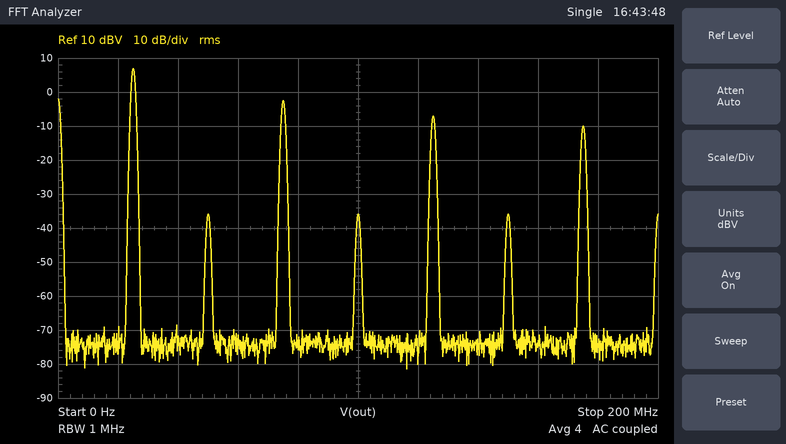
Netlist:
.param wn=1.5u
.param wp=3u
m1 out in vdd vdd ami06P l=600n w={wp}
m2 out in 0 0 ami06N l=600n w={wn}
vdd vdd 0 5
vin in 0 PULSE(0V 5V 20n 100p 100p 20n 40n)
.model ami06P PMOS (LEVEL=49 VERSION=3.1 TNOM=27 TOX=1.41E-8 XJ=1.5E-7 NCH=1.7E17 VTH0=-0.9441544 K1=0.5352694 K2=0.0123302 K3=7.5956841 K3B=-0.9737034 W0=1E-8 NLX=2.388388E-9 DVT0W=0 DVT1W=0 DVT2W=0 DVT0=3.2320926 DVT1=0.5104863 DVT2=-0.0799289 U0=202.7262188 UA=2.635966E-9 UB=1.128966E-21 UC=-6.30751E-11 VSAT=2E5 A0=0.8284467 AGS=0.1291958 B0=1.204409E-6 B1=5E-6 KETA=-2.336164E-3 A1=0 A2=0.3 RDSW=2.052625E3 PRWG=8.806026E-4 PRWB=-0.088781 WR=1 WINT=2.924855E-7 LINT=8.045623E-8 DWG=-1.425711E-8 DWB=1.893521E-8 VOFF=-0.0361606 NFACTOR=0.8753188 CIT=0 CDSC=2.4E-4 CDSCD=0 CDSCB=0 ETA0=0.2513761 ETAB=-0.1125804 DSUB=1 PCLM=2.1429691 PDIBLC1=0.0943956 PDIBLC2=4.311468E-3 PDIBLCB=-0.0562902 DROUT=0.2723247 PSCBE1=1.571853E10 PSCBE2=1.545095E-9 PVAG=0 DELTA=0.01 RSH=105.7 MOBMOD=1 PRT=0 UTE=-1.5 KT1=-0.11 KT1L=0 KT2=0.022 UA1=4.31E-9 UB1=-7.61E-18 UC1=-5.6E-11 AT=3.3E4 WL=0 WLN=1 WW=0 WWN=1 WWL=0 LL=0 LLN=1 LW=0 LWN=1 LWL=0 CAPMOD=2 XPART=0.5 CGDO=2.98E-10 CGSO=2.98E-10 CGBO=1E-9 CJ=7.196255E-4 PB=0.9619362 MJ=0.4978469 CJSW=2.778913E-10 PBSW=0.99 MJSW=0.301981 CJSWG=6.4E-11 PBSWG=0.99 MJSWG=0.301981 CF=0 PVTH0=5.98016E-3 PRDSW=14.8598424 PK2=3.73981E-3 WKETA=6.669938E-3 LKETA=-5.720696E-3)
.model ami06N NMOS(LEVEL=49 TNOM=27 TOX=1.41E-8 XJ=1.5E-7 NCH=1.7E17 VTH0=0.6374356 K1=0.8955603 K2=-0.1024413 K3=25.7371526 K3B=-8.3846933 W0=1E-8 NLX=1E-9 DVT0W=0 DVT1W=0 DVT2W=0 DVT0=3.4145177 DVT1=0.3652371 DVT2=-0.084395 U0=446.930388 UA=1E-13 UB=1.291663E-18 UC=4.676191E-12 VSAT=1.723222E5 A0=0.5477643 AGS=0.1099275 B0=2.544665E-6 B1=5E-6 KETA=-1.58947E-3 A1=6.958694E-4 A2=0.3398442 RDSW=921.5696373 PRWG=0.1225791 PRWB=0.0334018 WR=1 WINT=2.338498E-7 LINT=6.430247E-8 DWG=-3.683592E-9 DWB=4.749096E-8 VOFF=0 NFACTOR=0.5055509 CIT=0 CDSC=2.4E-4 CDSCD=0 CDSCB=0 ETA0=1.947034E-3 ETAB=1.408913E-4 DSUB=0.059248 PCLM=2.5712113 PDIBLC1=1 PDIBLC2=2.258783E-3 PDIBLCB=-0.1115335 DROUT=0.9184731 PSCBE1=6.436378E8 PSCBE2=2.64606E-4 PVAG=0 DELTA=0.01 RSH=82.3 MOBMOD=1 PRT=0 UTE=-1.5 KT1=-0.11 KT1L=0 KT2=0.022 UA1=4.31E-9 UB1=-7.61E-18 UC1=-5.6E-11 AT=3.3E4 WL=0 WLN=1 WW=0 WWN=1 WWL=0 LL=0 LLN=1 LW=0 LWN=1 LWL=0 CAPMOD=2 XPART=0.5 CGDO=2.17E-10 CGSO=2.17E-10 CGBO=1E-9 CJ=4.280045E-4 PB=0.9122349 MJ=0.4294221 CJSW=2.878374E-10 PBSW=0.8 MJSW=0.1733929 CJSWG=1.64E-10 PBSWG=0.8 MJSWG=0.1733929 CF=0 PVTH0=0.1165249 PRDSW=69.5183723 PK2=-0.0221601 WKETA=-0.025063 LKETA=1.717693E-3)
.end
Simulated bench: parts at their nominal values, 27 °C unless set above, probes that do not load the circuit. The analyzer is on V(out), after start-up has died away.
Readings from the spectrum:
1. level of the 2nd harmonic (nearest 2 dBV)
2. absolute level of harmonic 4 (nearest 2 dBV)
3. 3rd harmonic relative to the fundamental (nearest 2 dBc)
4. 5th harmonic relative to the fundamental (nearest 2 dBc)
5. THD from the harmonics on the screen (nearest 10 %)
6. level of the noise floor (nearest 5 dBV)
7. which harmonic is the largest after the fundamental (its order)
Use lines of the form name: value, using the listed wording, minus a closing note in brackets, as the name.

level of the 2nd harmonic: -36 dBV
absolute level of harmonic 4: -36 dBV
3rd harmonic relative to the fundamental: -10 dBc
5th harmonic relative to the fundamental: -14 dBc
THD from the harmonics on the screen: 40 %
level of the noise floor: -75 dBV
which harmonic is the largest after the fundamental: 3
